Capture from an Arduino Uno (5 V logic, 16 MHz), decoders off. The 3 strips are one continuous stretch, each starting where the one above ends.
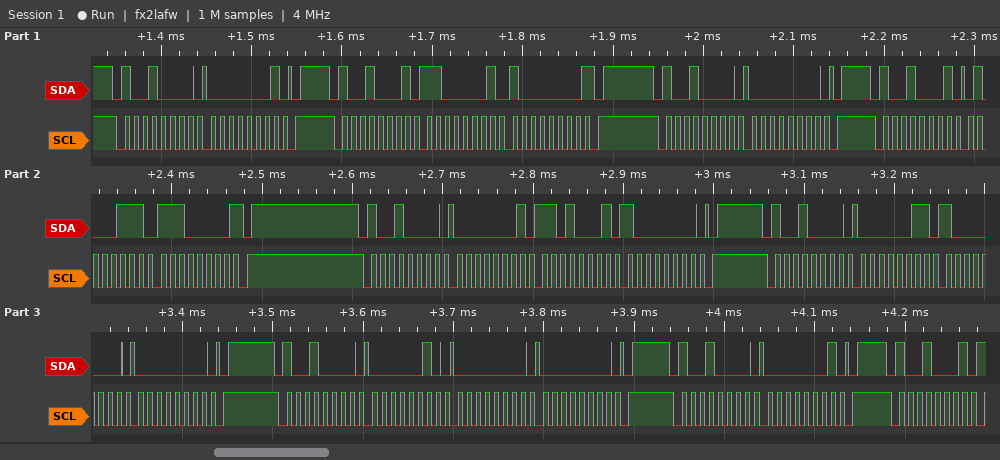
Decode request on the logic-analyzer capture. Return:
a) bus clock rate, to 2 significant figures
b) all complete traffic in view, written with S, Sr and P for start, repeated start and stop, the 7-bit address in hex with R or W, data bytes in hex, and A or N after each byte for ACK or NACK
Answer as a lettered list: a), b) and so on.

a) 100 kHz
b) S 48W A 01 A P S 48R A C1 A 80 N P S 48W A 00 A P S 48R A 47 A E0 N P S 48W A 01 A D1 A 80 A P S 48W A 03 A 80 A 00 A P S 48W A 02 A 00 A 00 A P S 48W A 01 A P S 48R A
